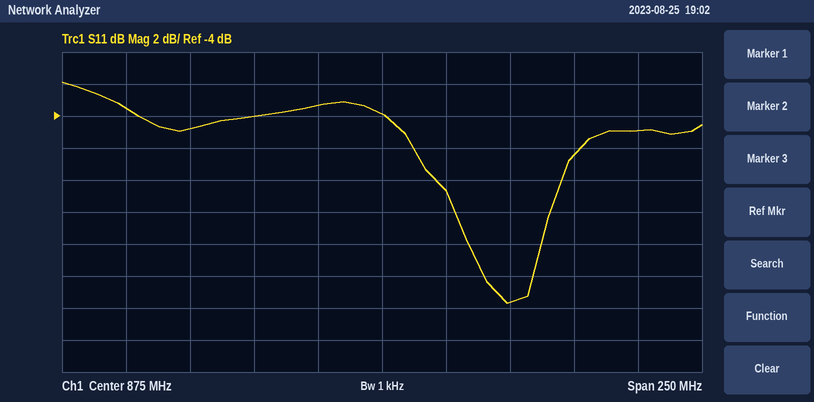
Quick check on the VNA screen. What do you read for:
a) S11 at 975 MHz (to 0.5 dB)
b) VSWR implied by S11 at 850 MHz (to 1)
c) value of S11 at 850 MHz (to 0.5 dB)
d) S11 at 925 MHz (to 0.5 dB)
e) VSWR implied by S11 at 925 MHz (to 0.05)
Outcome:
-5.0 dB
5
-3.5 dB
-15.5 dB
1.40
